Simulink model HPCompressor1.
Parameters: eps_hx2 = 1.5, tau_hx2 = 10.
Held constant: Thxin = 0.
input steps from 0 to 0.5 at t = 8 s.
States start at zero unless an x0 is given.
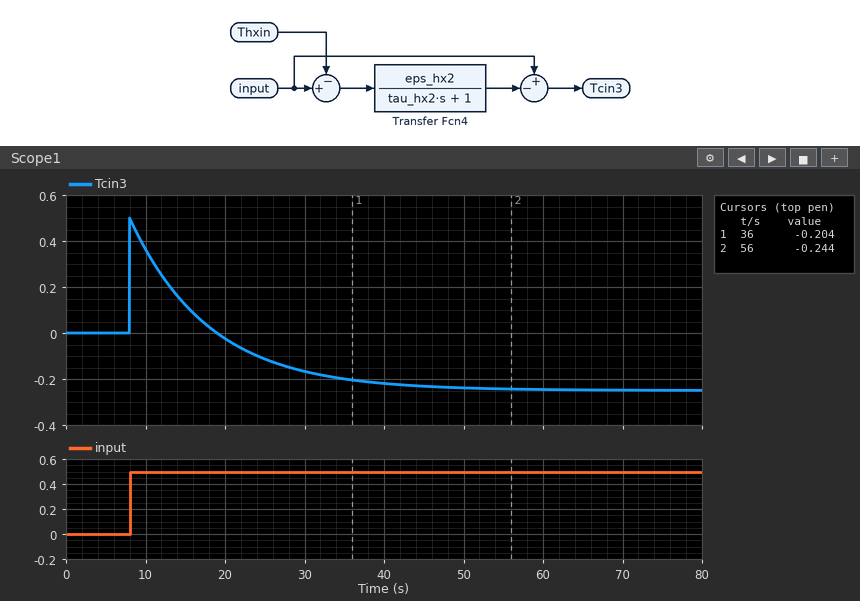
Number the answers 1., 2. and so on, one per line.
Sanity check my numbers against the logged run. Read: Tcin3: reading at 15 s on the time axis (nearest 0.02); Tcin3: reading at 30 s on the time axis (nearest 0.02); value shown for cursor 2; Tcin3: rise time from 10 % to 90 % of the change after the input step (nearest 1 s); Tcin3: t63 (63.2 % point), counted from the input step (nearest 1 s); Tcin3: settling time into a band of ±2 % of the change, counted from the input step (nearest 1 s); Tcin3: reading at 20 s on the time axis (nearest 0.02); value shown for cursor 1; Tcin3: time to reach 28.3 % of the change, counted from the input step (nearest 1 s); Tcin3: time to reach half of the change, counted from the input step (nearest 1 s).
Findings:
1. 0.12
2. -0.16
3. -0.244
4. 22 s
5. 21 s
6. 50 s
7. -0.02
8. -0.204
9. 14 s
10. 18 s
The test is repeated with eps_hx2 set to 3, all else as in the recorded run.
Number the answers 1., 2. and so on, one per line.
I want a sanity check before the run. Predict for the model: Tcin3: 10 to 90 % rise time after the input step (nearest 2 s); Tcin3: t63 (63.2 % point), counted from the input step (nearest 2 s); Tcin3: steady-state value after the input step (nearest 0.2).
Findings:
1. 22 s
2. 14 s
3. -1.0
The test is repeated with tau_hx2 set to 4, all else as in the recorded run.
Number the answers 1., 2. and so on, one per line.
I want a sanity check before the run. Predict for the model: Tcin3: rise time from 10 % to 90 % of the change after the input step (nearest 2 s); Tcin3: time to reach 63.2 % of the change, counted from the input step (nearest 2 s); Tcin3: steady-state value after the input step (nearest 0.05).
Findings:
1. 8 s
2. 8 s
3. -0.25
